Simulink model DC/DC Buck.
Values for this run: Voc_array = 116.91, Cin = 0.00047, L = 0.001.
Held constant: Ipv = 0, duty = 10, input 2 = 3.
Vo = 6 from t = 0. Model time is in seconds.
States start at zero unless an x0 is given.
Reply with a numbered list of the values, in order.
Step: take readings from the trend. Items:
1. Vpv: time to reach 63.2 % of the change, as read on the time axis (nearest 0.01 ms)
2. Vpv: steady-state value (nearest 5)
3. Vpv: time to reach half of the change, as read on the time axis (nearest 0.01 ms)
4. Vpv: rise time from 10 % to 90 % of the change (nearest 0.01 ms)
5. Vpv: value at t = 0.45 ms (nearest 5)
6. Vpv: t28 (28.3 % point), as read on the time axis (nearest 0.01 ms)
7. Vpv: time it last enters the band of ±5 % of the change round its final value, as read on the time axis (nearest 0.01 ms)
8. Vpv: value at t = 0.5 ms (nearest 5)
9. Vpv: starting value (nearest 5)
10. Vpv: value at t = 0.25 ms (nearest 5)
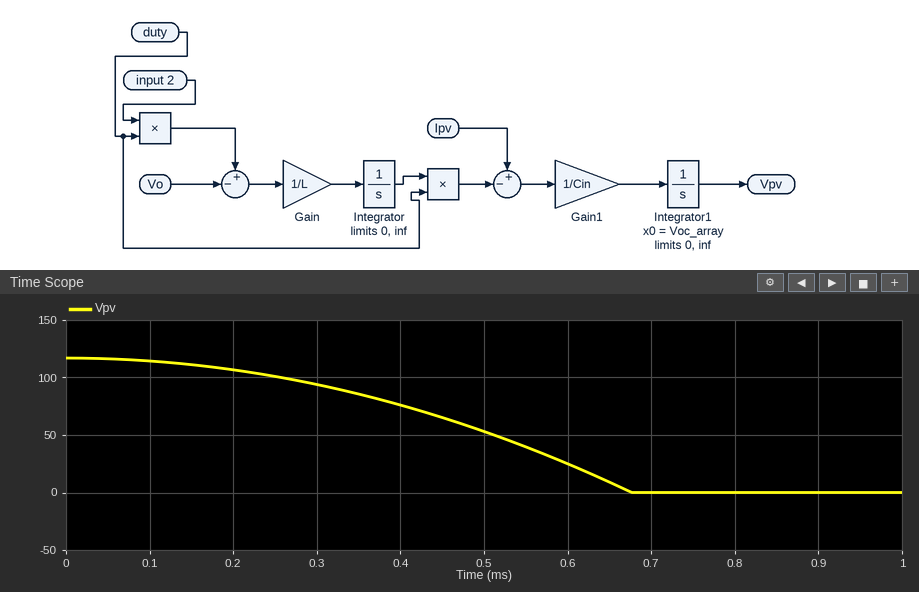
1. 0.54 ms
2. 0
3. 0.48 ms
4. 0.43 ms
5. 65
6. 0.36 ms
7. 0.66 ms
8. 55
9. 115
10. 100
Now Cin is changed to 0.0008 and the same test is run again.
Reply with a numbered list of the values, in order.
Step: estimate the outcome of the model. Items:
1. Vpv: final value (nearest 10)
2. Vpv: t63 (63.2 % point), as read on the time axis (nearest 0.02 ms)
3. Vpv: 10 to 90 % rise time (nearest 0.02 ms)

1. 0
2. 0.70 ms
3. 0.56 ms
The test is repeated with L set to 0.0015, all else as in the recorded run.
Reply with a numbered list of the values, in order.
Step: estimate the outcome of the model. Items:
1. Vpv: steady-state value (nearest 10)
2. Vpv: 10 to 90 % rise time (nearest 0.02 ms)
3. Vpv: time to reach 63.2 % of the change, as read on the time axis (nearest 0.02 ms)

1. 0
2. 0.52 ms
3. 0.66 ms
